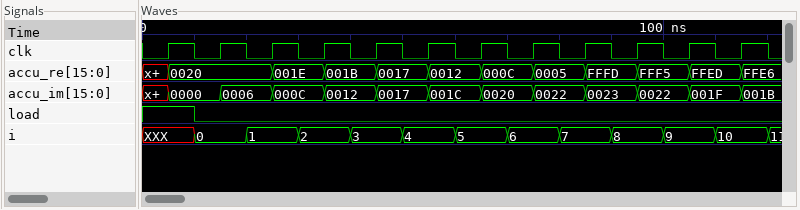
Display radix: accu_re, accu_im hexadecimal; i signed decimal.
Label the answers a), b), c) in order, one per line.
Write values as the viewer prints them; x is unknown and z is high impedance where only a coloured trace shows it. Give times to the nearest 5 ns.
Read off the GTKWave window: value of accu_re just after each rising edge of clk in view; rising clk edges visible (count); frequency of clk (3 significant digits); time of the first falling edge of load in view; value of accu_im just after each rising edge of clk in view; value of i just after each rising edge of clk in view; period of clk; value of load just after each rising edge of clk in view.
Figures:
a) 0020, 0020, 001E, 001B, 0017, 0012, 000C, 0005, FFFD, FFF5, FFED, FFE6
b) 12
c) 100 MHz
d) 10 ns
e) 0000, 0006, 000C, 0012, 0017, 001C, 0020, 0022, 0023, 0022, 001F, 001B
f) XXX, 0, 1, 2, 3, 4, 5, 6, 7, 8, 9, 10
g) 10 ns
h) 1 0 0 0 0 0 0 0 0 0 0 0
